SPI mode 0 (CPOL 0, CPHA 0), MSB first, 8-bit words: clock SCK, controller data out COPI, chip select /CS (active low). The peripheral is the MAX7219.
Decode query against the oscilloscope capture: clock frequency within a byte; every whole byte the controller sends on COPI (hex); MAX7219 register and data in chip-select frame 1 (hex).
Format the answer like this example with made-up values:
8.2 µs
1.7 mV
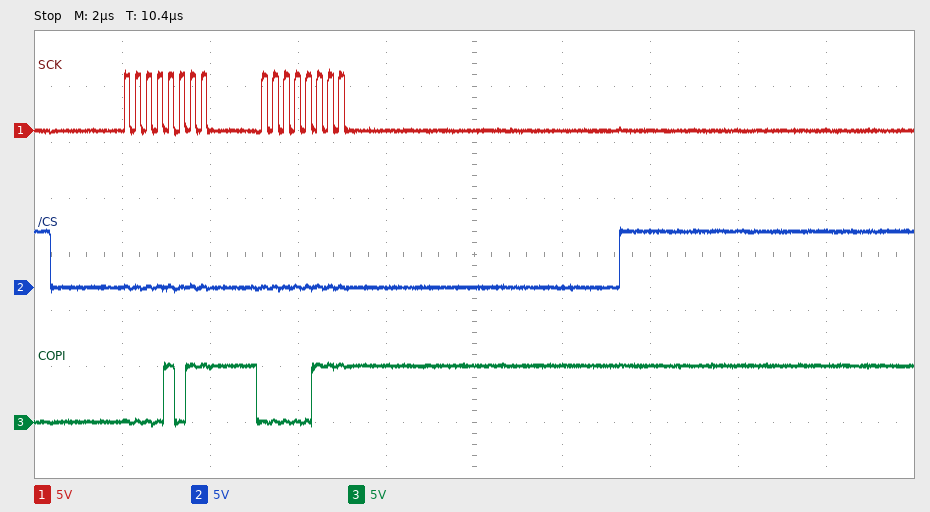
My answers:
4 MHz
0B 07
register 0xB, data 0x07
